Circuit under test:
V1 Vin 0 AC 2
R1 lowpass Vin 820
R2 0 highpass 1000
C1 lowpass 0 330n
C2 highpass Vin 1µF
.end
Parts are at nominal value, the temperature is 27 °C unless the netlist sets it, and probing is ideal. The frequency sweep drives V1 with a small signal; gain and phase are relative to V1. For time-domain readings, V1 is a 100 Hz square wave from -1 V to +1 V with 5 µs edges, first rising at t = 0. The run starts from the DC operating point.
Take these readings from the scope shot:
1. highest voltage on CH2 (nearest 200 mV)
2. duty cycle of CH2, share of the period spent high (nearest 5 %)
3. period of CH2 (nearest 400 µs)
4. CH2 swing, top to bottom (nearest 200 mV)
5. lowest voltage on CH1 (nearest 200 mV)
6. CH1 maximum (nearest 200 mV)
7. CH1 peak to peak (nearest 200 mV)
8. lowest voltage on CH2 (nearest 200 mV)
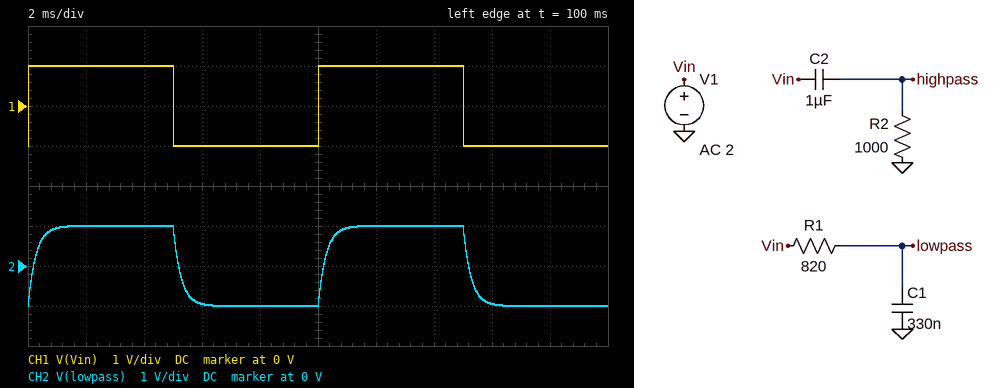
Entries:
1.0 V
50 %
10.0 ms
2.0 V
-1.0 V
1.0 V
2.0 V
-1.0 V
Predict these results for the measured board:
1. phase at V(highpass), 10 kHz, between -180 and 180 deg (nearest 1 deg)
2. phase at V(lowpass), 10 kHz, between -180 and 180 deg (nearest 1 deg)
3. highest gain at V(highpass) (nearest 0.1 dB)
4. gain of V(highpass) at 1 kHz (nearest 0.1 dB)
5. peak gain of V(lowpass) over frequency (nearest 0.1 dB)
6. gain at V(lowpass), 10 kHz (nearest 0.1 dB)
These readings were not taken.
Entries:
1 deg
-87 deg
0 dB
-0.1 dB
0 dB
-24.6 dB
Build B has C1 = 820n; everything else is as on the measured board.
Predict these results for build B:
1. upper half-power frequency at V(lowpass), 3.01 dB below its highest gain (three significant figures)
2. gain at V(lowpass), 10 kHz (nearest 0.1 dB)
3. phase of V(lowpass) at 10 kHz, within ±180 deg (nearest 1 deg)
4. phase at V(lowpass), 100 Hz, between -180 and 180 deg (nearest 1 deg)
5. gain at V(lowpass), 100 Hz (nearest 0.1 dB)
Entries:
237 Hz
-32.5 dB
-89 deg
-23 deg
-0.7 dB
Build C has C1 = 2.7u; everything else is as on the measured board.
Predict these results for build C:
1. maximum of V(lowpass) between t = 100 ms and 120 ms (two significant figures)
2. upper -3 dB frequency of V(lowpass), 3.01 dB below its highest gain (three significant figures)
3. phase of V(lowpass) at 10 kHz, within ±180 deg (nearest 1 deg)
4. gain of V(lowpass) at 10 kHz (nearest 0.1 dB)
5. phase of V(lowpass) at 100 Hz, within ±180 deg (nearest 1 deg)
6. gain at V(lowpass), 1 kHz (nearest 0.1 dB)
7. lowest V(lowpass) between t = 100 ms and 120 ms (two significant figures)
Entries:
810 mV
71.9 Hz
-90 deg
-42.9 dB
-54 deg
-22.9 dB
-810 mV
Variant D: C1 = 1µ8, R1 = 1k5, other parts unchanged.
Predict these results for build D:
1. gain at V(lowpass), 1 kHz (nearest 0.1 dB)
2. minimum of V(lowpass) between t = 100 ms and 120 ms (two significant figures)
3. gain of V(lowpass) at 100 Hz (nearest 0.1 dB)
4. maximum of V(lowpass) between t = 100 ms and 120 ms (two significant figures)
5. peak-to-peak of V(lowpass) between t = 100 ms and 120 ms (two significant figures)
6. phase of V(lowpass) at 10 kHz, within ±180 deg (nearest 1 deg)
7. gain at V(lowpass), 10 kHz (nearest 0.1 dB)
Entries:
-24.6 dB
-730 mV
-5.9 dB
730 mV
1.5 V
-90 deg
-44.6 dB
